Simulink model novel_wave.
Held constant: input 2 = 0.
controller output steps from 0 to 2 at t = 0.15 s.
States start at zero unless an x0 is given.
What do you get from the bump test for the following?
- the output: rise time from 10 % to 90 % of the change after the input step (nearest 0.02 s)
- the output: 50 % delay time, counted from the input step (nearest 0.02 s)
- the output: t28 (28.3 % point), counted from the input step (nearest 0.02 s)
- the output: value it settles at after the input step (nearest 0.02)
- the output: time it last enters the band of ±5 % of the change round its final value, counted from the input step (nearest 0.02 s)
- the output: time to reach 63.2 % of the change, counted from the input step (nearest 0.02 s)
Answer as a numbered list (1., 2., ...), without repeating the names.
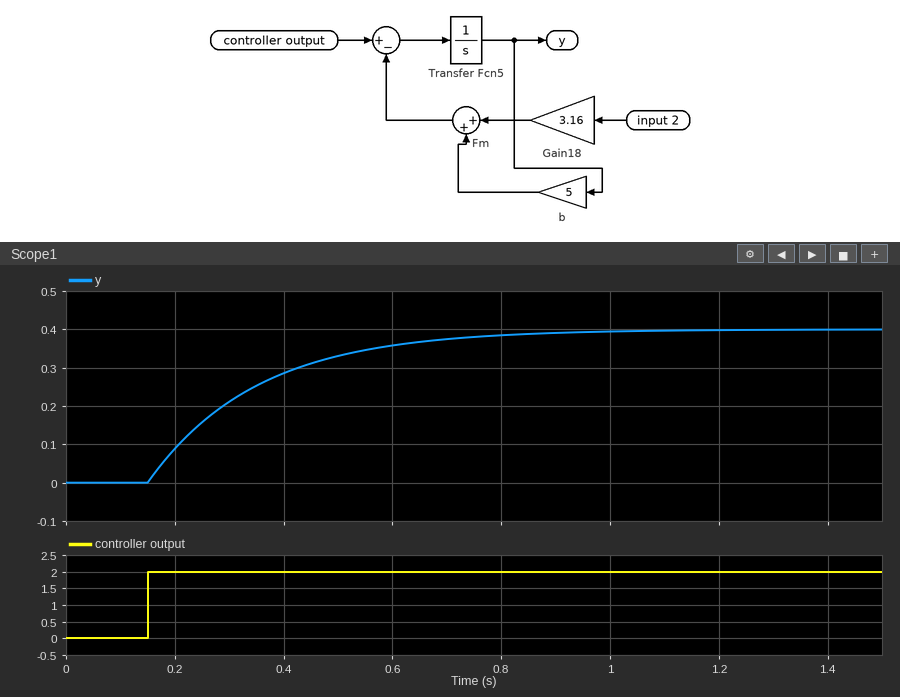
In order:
1. 0.44 s
2. 0.14 s
3. 0.06 s
4. 0.40
5. 0.60 s
6. 0.20 s
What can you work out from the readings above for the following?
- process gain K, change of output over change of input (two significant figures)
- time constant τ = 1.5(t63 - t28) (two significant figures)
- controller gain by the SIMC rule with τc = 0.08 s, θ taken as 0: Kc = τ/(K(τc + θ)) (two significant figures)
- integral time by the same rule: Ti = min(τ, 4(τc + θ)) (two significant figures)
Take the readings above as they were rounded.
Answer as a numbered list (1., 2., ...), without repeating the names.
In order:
1. 0.20
2. 0.21 s
3. 13
4. 0.21 s
